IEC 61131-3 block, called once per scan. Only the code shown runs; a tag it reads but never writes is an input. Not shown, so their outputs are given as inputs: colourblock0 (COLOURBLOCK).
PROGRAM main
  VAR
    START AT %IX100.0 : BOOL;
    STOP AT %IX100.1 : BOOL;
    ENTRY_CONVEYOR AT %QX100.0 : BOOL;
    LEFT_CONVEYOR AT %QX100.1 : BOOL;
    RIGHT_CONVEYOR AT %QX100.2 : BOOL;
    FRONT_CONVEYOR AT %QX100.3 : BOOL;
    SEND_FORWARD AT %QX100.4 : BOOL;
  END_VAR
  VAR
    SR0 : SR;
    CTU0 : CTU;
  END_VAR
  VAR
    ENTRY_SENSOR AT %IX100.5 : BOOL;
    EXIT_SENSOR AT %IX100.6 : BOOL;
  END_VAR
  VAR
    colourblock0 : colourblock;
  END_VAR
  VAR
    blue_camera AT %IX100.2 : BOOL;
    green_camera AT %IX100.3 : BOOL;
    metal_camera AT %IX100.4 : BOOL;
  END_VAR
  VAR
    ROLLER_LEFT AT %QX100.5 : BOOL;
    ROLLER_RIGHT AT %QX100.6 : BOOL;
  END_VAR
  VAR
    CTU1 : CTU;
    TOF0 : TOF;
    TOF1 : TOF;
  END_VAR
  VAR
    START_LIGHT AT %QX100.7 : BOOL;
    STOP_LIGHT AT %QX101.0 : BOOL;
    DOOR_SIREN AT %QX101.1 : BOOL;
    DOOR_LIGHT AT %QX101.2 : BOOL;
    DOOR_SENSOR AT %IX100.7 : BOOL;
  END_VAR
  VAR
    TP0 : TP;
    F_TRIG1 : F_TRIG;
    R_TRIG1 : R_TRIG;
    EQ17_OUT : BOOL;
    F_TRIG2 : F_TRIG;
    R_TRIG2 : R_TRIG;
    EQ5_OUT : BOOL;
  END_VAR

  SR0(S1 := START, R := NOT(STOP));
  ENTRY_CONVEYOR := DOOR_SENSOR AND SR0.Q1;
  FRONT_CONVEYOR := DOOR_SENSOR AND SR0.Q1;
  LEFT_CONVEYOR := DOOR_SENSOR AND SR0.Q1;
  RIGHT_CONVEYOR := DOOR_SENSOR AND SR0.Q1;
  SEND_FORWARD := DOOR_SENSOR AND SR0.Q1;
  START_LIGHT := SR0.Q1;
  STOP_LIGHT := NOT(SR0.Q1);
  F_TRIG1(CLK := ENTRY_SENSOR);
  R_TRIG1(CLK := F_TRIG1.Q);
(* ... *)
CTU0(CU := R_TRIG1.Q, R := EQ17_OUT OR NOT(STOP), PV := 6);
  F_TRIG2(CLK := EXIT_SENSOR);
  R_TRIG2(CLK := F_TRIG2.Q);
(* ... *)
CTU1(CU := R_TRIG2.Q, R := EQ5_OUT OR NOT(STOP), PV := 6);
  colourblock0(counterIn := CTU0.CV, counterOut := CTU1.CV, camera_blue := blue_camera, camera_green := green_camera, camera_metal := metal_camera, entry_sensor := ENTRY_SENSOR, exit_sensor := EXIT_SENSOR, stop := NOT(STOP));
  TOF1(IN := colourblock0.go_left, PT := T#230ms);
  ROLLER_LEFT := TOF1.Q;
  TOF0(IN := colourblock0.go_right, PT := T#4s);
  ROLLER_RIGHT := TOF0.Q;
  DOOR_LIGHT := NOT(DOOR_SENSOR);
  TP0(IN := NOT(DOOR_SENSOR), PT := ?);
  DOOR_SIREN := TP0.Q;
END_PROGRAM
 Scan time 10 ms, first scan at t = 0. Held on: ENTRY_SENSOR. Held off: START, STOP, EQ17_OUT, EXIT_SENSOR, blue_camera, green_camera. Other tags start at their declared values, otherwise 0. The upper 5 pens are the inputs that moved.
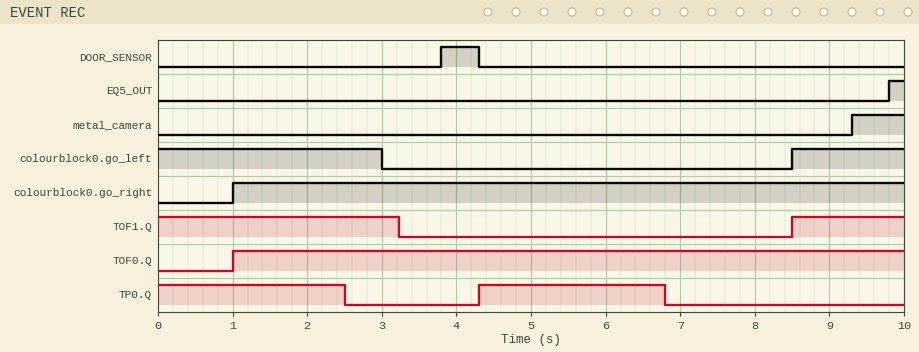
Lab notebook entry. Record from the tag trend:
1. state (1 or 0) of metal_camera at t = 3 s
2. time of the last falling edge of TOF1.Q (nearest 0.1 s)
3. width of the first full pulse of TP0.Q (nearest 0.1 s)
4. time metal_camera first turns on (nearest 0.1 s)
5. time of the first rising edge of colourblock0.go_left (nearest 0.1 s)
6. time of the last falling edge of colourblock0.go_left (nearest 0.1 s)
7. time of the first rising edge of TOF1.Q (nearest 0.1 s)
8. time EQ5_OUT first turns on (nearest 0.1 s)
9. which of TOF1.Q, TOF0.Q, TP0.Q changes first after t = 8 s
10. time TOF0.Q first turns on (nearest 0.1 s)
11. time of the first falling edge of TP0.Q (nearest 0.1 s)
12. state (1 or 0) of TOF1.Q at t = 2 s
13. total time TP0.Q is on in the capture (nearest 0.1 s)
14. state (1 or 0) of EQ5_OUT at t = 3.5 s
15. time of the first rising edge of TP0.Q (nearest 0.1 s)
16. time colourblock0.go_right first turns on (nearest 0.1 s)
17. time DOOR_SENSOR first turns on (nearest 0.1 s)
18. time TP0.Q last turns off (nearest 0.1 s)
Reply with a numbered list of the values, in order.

1. 0
2. 3.2 s
3. 2.5 s
4. 9.3 s
5. 8.5 s
6. 3.0 s
7. 8.5 s
8. 9.8 s
9. TOF1.Q
10. 1.0 s
11. 2.5 s
12. 1
13. 5.0 s
14. 0
15. 4.3 s
16. 1.0 s
17. 3.8 s
18. 6.8 s
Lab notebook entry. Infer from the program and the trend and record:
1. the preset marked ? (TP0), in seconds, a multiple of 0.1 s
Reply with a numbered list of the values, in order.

1. 2.5 s
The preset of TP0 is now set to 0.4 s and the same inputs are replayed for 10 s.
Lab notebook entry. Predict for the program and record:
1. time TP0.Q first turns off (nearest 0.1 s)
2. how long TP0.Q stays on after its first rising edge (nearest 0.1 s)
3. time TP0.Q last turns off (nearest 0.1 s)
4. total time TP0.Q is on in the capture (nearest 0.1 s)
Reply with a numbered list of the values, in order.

1. 0.4 s
2. 0.4 s
3. 4.7 s
4. 0.8 s
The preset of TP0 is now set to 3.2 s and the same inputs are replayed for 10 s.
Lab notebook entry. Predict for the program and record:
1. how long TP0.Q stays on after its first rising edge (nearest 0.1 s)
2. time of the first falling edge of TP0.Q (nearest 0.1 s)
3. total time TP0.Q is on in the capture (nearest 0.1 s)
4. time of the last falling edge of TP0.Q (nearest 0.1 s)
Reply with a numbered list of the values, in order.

1. 3.2 s
2. 3.2 s
3. 6.4 s
4. 7.5 s
